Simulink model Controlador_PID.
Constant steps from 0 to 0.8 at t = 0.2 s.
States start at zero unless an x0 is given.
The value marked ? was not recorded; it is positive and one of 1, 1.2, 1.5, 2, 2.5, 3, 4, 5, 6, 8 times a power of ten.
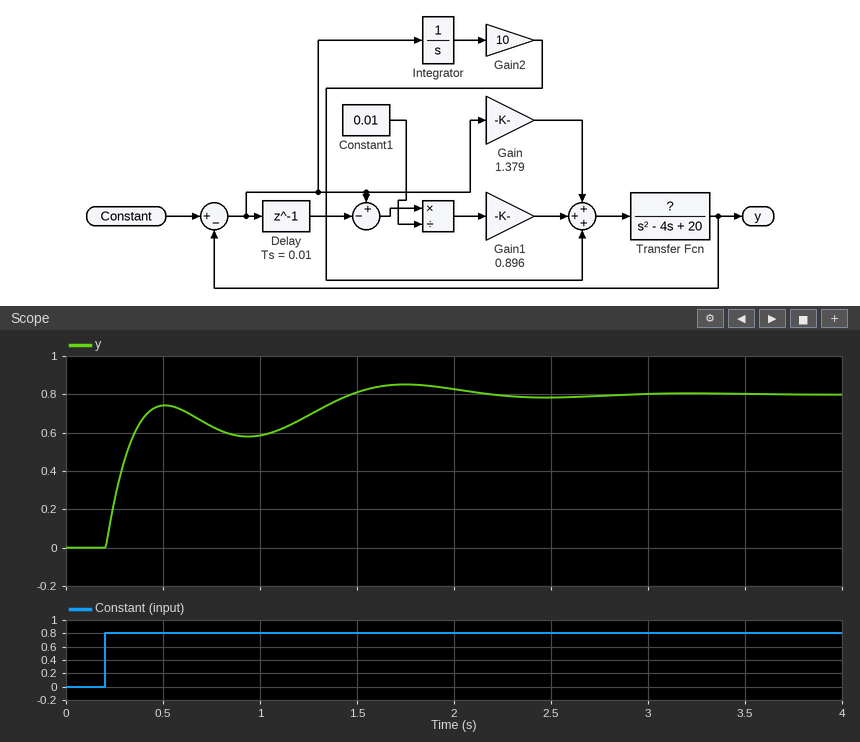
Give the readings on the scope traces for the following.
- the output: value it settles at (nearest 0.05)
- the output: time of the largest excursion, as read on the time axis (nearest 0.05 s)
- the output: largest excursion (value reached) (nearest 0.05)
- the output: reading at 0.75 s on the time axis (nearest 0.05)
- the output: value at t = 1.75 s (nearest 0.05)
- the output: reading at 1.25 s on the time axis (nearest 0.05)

0.80
1.75 s
0.85
0.65
0.85
0.70
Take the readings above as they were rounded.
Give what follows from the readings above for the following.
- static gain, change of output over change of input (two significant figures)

1.0
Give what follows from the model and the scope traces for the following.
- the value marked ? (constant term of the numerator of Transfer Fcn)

8
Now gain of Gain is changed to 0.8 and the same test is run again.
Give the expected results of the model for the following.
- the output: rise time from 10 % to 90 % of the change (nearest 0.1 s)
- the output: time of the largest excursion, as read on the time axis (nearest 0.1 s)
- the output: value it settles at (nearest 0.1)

1.1 s
1.8 s
0.8
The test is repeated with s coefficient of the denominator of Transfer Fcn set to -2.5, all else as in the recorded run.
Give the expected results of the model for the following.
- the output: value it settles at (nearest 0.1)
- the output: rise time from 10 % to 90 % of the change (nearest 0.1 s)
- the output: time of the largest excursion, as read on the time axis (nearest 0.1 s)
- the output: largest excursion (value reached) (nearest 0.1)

0.8
1.0 s
1.8 s
0.8
